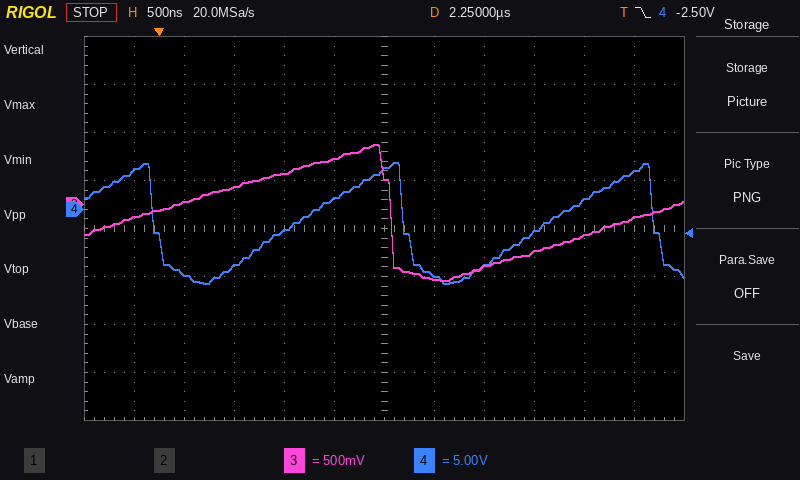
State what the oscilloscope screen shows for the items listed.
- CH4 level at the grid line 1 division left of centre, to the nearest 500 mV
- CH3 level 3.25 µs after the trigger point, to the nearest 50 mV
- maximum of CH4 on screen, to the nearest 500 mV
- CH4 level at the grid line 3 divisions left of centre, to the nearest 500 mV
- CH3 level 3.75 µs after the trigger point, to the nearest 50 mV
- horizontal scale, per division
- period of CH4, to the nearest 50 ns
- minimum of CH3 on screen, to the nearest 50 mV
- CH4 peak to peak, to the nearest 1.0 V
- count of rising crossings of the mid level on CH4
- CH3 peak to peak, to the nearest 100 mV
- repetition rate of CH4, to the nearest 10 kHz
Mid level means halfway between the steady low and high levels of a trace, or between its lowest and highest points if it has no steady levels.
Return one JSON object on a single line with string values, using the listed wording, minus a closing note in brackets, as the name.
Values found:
{"CH4 level at the grid line 1 division left of centre, to the nearest 500 mV": "1.0 V", "CH3 level 3.25 µs after the trigger point, to the nearest 50 mV": "-650 mV", "maximum of CH4 on screen, to the nearest 500 mV": "5.0 V", "CH4 level at the grid line 3 divisions left of centre, to the nearest 500 mV": "-6.0 V", "CH3 level 3.75 µs after the trigger point, to the nearest 50 mV": "-500 mV", "horizontal scale, per division": "500 ns", "period of CH4, to the nearest 50 ns": "2.50 µs", "minimum of CH3 on screen, to the nearest 50 mV": "-800 mV", "CH4 peak to peak, to the nearest 1.0 V": "13.0 V", "count of rising crossings of the mid level on CH4": "2", "CH3 peak to peak, to the nearest 100 mV": "1.40 V", "repetition rate of CH4, to the nearest 10 kHz": "400 kHz"}
